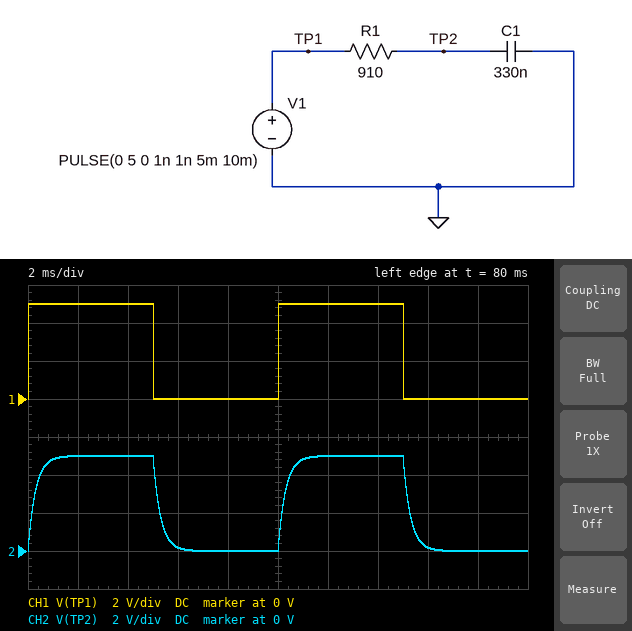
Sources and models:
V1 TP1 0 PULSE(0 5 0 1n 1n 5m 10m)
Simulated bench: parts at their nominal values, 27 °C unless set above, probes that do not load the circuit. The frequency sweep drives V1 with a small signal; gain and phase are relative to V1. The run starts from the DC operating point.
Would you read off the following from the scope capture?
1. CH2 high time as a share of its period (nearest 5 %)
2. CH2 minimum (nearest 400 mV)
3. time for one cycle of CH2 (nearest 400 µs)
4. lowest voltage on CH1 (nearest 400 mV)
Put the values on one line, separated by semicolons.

50 %; 0 V; 10.0 ms; 0 V
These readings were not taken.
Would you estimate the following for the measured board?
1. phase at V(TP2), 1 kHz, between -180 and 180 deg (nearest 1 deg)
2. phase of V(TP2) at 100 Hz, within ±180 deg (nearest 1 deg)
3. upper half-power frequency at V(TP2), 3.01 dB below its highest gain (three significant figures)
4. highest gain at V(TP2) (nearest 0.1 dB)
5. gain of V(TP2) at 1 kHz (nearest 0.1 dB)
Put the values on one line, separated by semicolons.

-62 deg; -11 deg; 530 Hz; 0 dB; -6.6 dB
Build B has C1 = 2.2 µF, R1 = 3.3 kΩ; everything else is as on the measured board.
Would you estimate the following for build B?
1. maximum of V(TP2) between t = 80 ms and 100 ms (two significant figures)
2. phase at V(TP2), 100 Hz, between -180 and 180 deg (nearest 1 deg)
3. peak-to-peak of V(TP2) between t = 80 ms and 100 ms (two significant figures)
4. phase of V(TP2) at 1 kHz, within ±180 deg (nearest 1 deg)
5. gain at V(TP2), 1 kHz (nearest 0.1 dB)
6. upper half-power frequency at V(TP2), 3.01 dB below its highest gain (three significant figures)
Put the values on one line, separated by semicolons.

3.3 V; -78 deg; 1.7 V; -89 deg; -33.2 dB; 21.9 Hz
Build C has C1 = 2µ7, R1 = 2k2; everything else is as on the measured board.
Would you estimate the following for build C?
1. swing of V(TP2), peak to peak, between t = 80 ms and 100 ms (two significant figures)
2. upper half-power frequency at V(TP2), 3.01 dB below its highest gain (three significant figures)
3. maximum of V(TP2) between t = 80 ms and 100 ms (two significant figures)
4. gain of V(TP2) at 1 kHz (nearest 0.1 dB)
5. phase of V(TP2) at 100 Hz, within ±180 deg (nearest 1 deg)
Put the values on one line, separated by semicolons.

2.0 V; 26.8 Hz; 3.5 V; -31.4 dB; -75 deg
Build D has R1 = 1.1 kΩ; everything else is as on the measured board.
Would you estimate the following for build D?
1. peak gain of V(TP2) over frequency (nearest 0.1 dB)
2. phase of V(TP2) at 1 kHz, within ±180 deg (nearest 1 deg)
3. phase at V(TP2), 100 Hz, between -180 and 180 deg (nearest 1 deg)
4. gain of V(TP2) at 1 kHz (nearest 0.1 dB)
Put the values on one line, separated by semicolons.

0 dB; -66 deg; -13 deg; -7.9 dB
